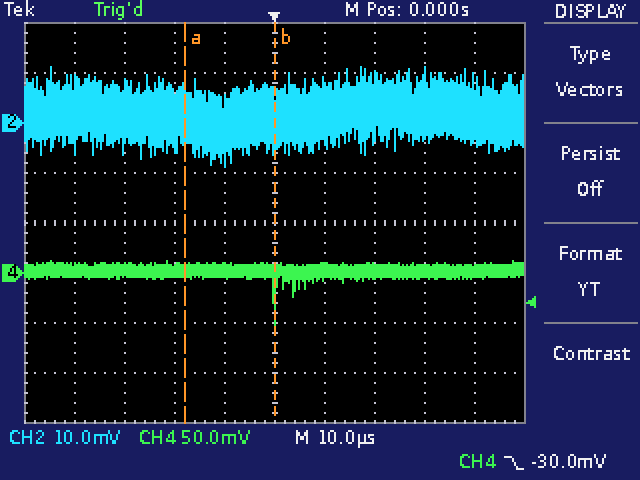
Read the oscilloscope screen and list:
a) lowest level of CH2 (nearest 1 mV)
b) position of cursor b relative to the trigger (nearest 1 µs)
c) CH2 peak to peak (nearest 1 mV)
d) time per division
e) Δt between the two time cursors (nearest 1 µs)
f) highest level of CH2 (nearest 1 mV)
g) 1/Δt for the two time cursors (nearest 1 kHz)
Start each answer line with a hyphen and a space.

- -9 mV
- 0 µs
- 20 mV
- 10 µs
- 18 µs
- 11 mV
- 56 kHz
